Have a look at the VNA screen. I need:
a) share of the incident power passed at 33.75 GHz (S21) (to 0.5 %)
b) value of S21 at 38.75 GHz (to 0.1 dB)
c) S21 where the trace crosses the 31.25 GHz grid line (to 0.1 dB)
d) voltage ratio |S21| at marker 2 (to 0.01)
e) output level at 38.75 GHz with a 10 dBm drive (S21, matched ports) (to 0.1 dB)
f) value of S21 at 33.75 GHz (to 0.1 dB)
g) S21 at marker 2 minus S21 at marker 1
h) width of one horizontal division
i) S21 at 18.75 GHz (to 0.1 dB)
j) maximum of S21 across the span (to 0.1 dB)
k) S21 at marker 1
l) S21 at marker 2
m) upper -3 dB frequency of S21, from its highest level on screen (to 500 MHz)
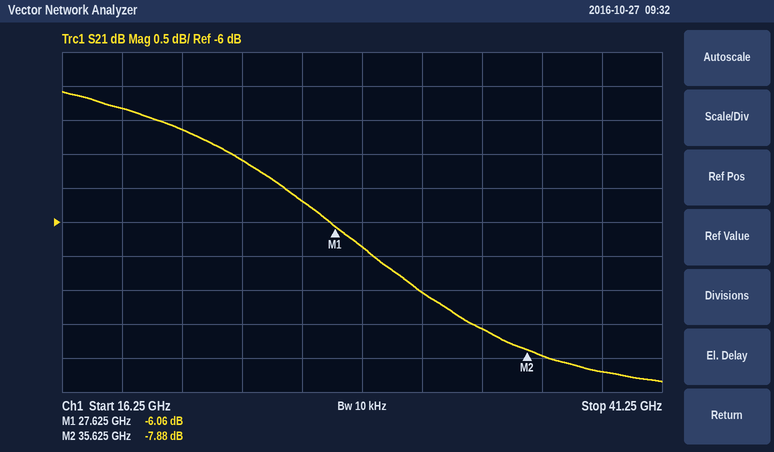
17.5 %
-8.2 dB
-7.0 dB
0.40
1.8 dBm
-7.6 dB
-1.82 dB
2.5 GHz
-4.3 dB
-4.1 dB
-6.06 dB
-7.88 dB
31.5 GHz
